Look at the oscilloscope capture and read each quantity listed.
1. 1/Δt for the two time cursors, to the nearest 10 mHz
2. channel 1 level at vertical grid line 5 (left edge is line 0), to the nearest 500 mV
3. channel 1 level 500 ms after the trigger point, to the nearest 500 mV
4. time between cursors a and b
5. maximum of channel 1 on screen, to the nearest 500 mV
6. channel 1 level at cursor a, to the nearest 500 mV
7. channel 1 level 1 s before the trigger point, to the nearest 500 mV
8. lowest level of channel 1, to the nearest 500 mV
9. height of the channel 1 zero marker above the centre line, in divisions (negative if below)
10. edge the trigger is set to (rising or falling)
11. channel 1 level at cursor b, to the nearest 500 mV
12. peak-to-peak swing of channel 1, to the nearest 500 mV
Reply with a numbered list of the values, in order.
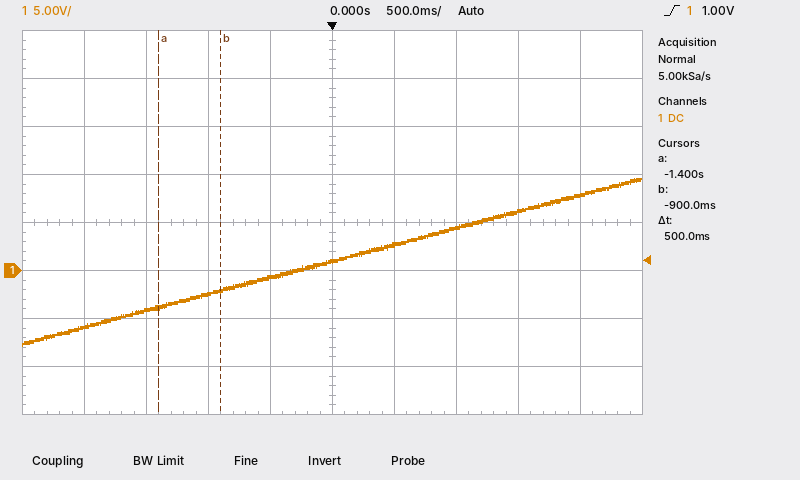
1. 2.00 Hz
2. 1.0 V
3. 2.5 V
4. 500 ms
5. 9.5 V
6. -4.0 V
7. -2.5 V
8. -8.0 V
9. -1.0 div
10. rising
11. -2.0 V
12. 17.5 V
